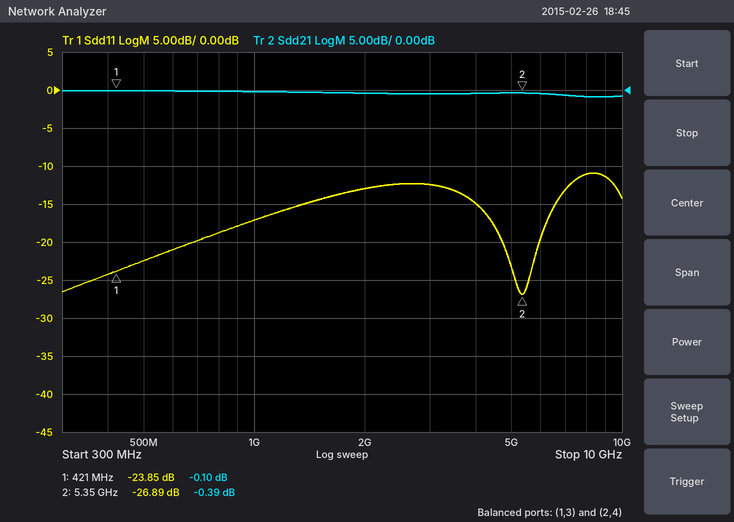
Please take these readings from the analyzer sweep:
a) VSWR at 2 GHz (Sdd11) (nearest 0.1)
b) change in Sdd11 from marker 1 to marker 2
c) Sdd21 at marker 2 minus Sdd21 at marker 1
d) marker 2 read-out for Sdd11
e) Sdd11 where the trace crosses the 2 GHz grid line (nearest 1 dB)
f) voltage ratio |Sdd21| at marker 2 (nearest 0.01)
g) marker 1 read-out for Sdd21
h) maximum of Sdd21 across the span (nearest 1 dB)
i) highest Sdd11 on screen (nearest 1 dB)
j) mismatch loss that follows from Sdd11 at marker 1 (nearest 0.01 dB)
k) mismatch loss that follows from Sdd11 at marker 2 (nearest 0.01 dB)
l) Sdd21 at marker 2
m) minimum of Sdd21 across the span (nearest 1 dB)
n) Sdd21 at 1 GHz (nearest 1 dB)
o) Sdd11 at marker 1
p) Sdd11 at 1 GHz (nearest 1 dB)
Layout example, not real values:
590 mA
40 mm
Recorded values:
1.6
-3.04 dB
-0.29 dB
-26.89 dB
-13 dB
0.96
-0.10 dB
0 dB
-11 dB
0.02 dB
0.01 dB
-0.39 dB
-1 dB
0 dB
-23.85 dB
-17 dB
